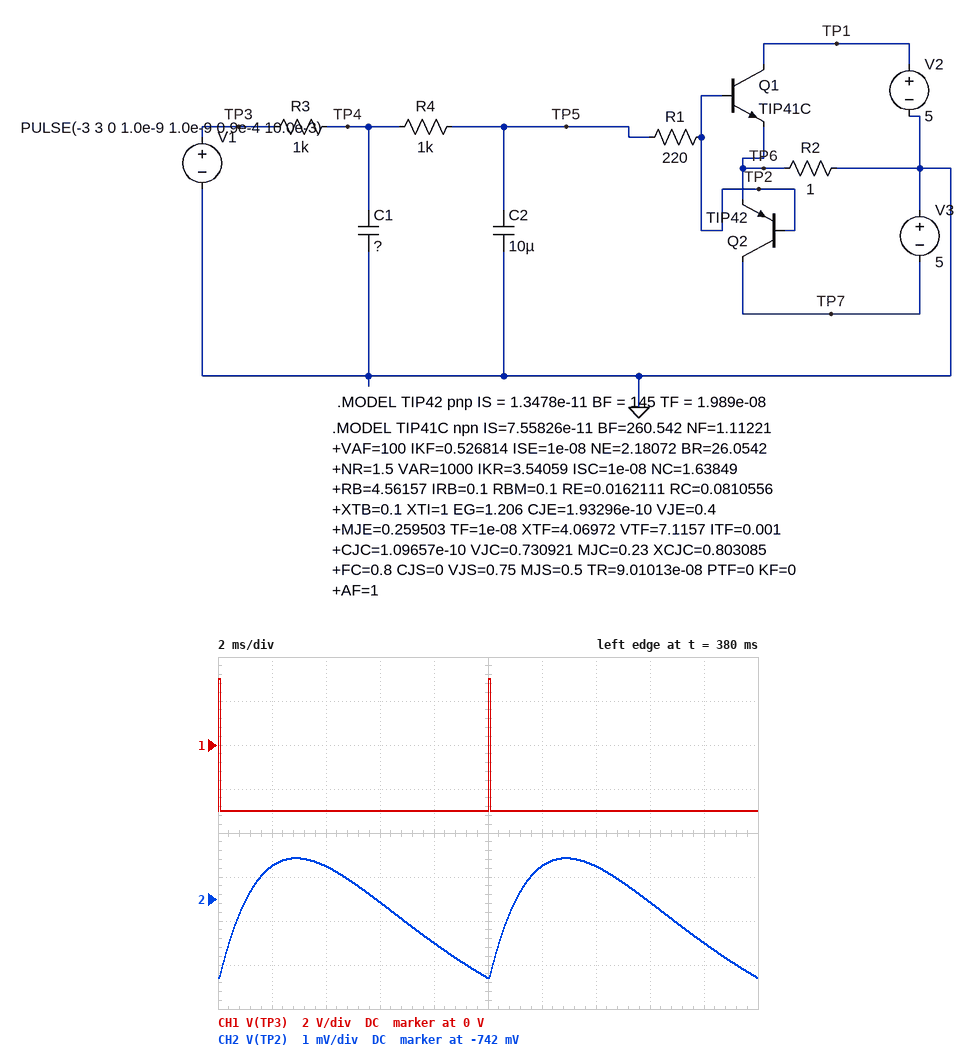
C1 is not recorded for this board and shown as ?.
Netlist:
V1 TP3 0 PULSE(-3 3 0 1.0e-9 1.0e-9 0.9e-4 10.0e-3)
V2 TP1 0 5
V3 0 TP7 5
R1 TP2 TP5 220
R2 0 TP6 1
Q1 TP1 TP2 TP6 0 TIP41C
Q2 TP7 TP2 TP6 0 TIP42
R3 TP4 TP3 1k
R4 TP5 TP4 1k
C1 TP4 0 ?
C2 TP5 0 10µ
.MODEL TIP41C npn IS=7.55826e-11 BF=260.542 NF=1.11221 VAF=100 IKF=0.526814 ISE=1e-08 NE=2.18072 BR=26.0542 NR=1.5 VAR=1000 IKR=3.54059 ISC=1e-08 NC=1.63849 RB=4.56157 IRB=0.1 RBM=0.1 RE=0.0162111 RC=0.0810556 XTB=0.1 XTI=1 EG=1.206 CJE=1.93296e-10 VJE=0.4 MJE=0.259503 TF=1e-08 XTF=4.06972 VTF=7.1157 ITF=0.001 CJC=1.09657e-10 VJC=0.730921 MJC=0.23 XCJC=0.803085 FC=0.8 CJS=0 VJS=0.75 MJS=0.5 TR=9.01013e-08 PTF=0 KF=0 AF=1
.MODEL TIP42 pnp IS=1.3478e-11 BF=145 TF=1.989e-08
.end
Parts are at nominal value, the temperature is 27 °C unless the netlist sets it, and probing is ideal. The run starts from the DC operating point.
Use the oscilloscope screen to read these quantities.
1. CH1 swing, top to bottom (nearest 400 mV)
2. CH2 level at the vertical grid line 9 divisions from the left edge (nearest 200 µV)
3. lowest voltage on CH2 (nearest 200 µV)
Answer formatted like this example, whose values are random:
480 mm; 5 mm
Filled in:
6.0 V; -743.0 mV; -743.8 mV
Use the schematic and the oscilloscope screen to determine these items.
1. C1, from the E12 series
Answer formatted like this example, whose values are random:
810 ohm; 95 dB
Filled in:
8.2 µF
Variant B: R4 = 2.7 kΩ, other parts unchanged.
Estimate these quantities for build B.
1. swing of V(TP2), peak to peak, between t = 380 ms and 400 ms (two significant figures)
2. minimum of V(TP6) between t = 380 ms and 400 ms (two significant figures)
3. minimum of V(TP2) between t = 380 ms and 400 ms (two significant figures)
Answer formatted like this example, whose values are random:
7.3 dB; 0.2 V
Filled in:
1.2 mV; -85 mV; -670 mV
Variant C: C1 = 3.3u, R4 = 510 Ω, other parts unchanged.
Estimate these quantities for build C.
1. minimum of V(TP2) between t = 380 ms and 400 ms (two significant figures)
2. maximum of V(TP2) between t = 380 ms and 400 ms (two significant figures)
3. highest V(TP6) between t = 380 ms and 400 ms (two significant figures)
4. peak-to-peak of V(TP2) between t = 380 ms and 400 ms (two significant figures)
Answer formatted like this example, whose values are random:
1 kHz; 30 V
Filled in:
-790 mV; -780 mV; -180 mV; 7.6 mV
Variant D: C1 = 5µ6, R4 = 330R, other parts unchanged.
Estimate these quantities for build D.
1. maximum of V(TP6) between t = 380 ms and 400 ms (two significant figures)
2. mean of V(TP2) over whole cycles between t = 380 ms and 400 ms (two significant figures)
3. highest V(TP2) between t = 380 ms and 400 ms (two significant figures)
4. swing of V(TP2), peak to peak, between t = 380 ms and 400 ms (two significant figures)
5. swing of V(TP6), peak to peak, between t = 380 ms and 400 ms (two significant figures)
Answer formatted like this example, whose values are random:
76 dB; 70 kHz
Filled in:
-200 mV; -810 mV; -800 mV; 7.2 mV; 6.4 mV
